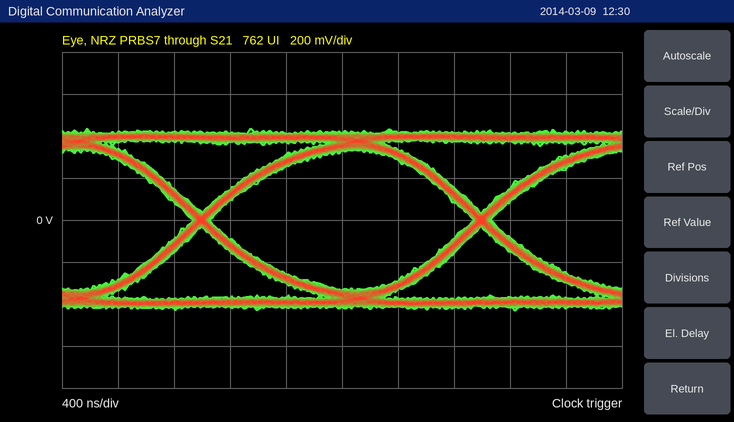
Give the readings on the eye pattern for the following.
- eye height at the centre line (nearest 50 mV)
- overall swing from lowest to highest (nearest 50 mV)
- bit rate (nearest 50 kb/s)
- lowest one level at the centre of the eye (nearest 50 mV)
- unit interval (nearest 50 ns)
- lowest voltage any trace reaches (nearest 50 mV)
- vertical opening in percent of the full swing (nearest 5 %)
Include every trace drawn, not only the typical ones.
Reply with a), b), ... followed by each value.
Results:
a) 650 mV
b) 850 mV
c) 500 kb/s
d) 350 mV
e) 2.00 µs
f) -450 mV
g) 75 %
